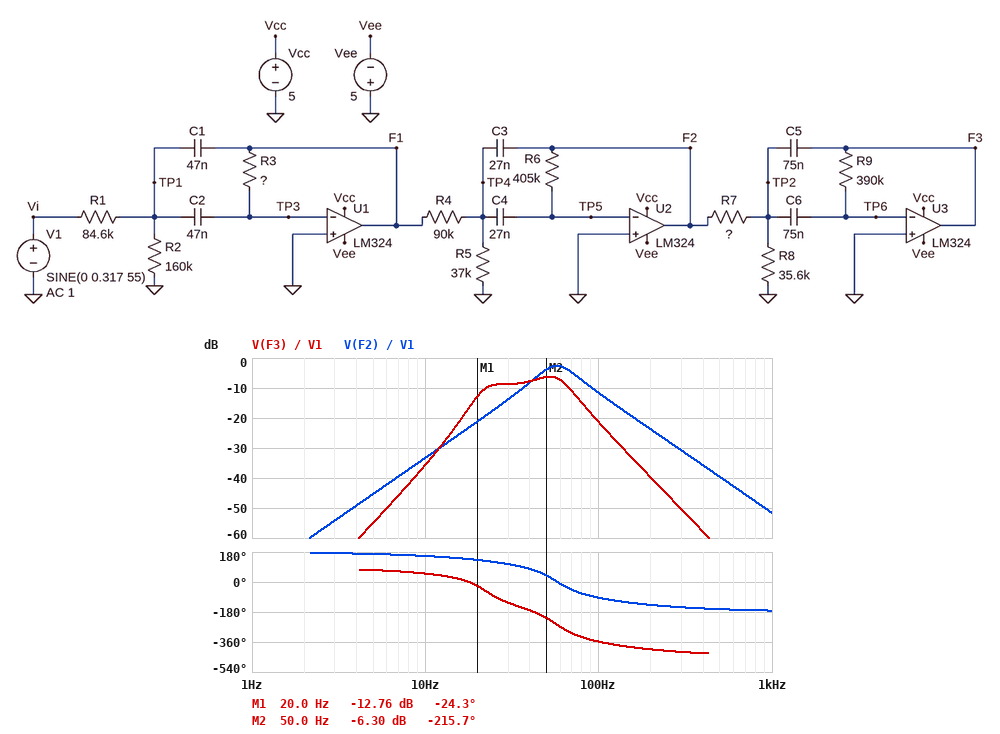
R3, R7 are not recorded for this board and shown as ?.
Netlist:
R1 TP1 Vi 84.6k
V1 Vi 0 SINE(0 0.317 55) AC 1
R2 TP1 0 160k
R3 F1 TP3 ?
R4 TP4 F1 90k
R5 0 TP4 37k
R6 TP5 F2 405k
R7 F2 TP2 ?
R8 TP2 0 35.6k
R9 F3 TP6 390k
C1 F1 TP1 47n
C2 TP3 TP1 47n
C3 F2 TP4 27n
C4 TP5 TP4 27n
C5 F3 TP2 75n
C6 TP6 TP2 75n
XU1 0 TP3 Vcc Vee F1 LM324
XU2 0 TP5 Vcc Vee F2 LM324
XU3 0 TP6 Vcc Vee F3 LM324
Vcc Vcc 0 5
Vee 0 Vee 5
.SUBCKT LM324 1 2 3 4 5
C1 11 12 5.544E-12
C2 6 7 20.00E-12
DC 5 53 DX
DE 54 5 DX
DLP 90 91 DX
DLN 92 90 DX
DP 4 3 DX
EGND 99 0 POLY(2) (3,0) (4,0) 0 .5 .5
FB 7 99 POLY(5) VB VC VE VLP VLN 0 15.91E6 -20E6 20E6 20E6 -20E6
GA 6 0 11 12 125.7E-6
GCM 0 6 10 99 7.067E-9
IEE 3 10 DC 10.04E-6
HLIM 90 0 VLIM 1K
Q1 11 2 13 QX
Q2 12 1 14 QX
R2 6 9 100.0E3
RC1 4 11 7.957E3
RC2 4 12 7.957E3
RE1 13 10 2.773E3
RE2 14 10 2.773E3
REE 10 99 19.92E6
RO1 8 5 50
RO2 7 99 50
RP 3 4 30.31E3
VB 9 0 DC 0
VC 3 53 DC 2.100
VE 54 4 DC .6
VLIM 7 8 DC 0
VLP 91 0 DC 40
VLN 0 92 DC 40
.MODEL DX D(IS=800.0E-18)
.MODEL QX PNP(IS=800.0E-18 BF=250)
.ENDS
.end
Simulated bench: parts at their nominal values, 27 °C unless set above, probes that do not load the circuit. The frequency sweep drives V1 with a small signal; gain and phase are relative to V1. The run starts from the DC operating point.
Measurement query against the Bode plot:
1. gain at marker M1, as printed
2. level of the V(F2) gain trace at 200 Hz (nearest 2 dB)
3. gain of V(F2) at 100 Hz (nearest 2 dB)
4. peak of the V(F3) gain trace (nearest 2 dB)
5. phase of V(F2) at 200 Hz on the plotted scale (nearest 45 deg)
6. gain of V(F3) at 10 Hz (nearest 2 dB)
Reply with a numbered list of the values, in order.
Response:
1. -12.76 dB
2. -24 dB
3. -12 dB
4. -6 dB
5. -135 deg
6. -36 dB
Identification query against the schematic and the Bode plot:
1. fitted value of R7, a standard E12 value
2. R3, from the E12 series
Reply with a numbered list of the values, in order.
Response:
1. 68 kΩ
2. 56 kΩ
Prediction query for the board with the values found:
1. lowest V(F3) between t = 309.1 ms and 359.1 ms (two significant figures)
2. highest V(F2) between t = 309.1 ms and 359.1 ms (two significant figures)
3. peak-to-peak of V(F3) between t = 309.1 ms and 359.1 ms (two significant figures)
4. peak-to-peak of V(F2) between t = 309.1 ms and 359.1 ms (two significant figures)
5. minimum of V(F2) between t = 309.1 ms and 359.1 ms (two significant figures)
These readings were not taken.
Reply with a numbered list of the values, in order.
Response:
1. -160 mV
2. 220 mV
3. 310 mV
4. 460 mV
5. -240 mV
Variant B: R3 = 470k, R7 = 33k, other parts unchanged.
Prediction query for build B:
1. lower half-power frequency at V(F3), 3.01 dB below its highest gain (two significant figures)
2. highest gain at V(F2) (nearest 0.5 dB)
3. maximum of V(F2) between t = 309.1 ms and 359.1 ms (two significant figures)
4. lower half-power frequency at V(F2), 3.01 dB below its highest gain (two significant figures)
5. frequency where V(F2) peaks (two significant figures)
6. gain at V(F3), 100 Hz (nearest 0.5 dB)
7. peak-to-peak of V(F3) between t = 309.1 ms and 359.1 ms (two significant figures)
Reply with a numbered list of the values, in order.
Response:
1. 22 Hz
2. 5.5 dB
3. 570 mV
4. 21 Hz
5. 52 Hz
6. -12.0 dB
7. 1.7 V
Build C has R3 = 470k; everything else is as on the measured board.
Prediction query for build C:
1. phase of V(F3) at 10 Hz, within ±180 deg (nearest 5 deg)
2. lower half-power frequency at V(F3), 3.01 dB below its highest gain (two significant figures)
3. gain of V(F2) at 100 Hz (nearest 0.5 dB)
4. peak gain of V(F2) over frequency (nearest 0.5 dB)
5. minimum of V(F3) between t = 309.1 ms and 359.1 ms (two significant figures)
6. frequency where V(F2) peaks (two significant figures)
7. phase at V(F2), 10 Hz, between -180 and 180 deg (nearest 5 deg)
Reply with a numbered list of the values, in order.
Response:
1. 45 deg
2. 19 Hz
3. -8.5 dB
4. 5.5 dB
5. -390 mV
6. 52 Hz
7. 150 deg
